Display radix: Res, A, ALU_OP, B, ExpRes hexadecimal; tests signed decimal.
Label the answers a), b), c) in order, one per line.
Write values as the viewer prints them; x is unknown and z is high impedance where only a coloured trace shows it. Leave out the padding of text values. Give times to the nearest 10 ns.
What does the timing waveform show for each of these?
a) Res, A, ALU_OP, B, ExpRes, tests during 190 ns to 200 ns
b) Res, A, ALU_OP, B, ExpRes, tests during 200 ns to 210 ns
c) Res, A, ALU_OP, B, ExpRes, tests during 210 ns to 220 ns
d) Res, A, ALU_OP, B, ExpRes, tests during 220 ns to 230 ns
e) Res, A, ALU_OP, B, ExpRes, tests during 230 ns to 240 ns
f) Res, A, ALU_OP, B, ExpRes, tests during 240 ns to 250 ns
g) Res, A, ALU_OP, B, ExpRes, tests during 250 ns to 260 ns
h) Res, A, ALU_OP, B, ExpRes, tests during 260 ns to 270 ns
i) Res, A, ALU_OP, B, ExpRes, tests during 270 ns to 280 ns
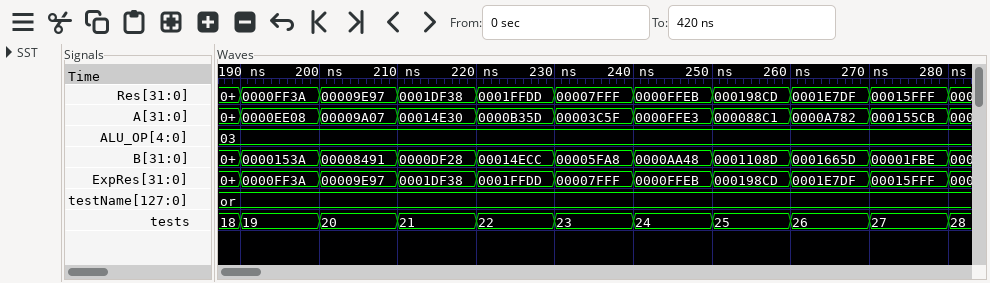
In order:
a) Res=0000FF3A, A=0000EE08, ALU_OP=03, B=0000153A, ExpRes=0000FF3A, tests=19
b) Res=00009E97, A=00009A07, ALU_OP=03, B=00008491, ExpRes=00009E97, tests=20
c) Res=0001DF38, A=00014E30, ALU_OP=03, B=0000DF28, ExpRes=0001DF38, tests=21
d) Res=0001FFDD, A=0000B35D, ALU_OP=03, B=00014ECC, ExpRes=0001FFDD, tests=22
e) Res=00007FFF, A=00003C5F, ALU_OP=03, B=00005FA8, ExpRes=00007FFF, tests=23
f) Res=0000FFEB, A=0000FFE3, ALU_OP=03, B=0000AA48, ExpRes=0000FFEB, tests=24
g) Res=000198CD, A=000088C1, ALU_OP=03, B=0001108D, ExpRes=000198CD, tests=25
h) Res=0001E7DF, A=0000A782, ALU_OP=03, B=0001665D, ExpRes=0001E7DF, tests=26
i) Res=00015FFF, A=000155CB, ALU_OP=03, B=00001FBE, ExpRes=00015FFF, tests=27
